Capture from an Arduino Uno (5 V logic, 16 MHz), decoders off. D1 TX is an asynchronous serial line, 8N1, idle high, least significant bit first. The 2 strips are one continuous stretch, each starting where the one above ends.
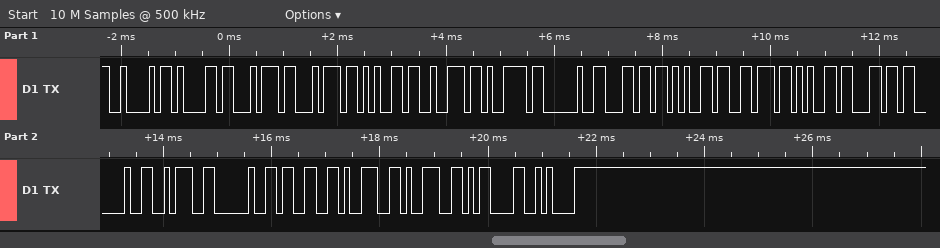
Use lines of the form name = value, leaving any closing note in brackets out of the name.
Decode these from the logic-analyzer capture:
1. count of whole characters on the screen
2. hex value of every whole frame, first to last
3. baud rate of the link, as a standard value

count of whole characters on the screen = 21
hex value of every whole frame, first to last = 42 61 74 74 65 72 79 20 6C 65 76 65 6C 20 3A 20 33 39 39 0D 0A
baud rate of the link, as a standard value = 9600 baud
